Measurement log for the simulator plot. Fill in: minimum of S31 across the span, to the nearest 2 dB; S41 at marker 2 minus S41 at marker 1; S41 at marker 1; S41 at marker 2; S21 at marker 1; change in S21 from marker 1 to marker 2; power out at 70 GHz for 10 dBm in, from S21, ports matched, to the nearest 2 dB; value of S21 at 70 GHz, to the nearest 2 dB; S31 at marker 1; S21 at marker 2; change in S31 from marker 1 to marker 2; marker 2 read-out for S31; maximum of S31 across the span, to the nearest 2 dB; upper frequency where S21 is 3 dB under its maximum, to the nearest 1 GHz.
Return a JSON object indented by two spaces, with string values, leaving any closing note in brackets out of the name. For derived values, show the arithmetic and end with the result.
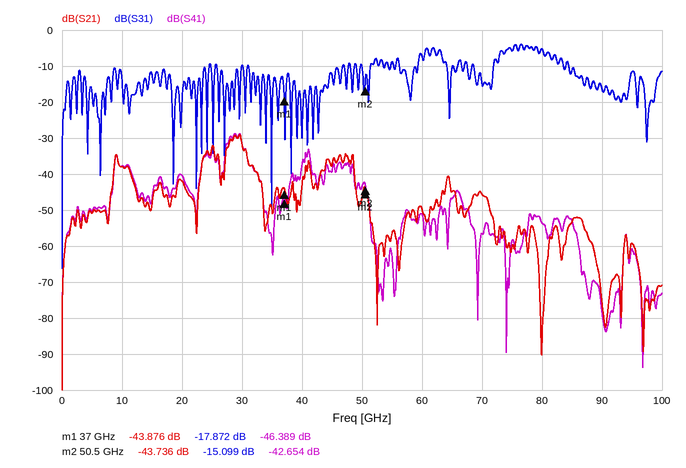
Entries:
{
  "minimum of S31 across the span, to the nearest 2 dB": "-66 dB",
  "S41 at marker 2 minus S41 at marker 1": "-42.654 − (-46.389) = 3.735 dB",
  "S41 at marker 1": "-46.389 dB",
  "S41 at marker 2": "-42.654 dB",
  "S21 at marker 1": "-43.876 dB",
  "change in S21 from marker 1 to marker 2": "-43.736 − (-43.876) = 0.140 dB",
  "power out at 70 GHz for 10 dBm in, from S21, ports matched, to the nearest 2 dB": "10 dBm + (-46 dB) = -36 dBm",
  "value of S21 at 70 GHz, to the nearest 2 dB": "-46 dB",
  "S31 at marker 1": "-17.872 dB",
  "S21 at marker 2": "-43.736 dB",
  "change in S31 from marker 1 to marker 2": "-15.099 − (-17.872) = 2.773 dB",
  "marker 2 read-out for S31": "-15.099 dB",
  "maximum of S31 across the span, to the nearest 2 dB": "-4 dB",
  "upper frequency where S21 is 3 dB under its maximum, to the nearest 1 GHz": "30 GHz"
}
